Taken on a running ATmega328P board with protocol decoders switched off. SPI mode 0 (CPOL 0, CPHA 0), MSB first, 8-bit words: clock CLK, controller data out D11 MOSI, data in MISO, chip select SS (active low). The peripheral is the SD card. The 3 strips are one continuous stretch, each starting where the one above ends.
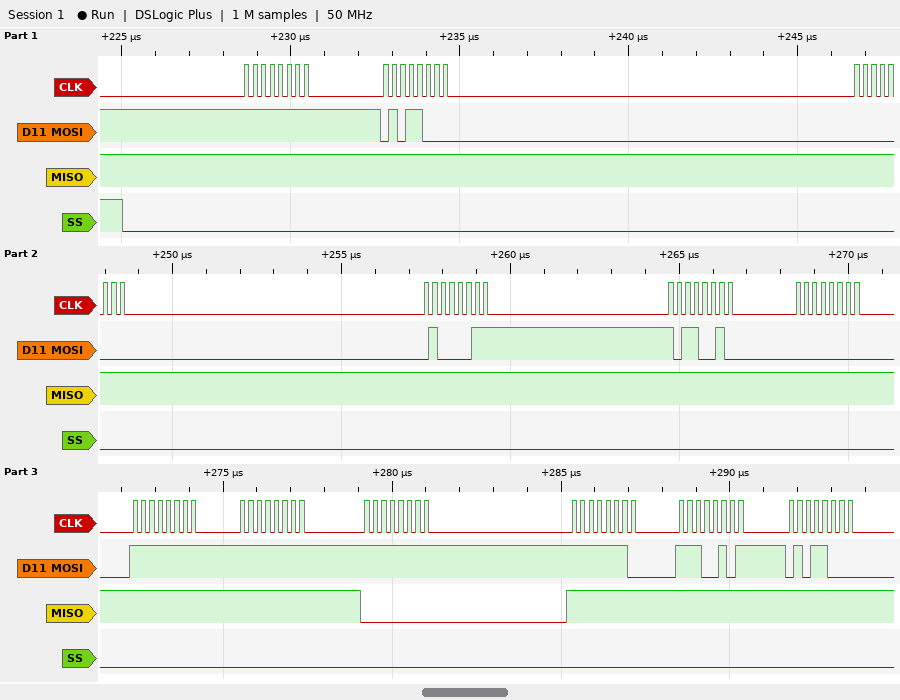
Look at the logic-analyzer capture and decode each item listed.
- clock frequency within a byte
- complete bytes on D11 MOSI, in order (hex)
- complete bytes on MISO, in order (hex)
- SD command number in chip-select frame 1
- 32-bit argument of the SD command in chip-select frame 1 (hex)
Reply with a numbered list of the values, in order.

1. 4 MHz
2. FF 58 00 43 B2 00 FF FF FF FE E5 58
3. FF FF FF FF FF FF FF FF 00 FF FF FF
4. CMD24
5. 0x0043B200
